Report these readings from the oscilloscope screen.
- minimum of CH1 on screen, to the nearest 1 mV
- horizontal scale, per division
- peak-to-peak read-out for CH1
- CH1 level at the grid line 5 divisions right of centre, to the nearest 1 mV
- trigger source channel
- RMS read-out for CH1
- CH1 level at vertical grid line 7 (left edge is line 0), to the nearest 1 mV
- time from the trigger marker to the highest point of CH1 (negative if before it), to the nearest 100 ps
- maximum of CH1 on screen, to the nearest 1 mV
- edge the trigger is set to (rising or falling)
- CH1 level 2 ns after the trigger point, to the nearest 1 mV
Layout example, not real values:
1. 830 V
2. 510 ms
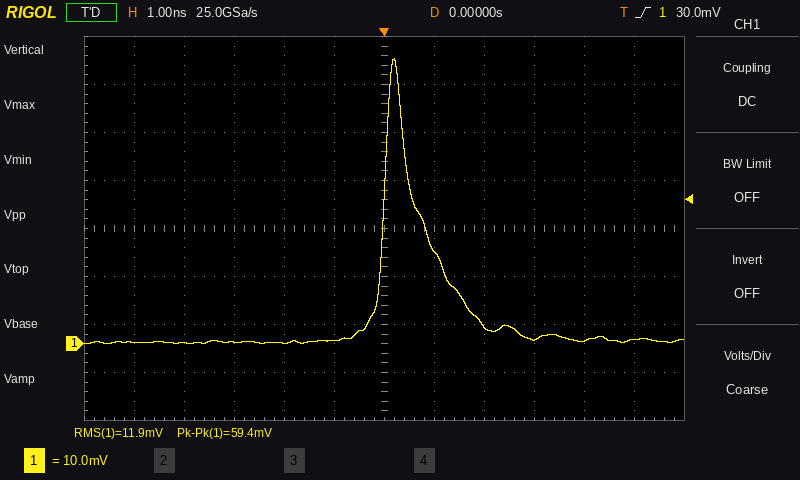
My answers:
1. 0 mV
2. 1 ns
3. 59.4 mV
4. 1 mV
5. CH1
6. 11.9 mV
7. 19 mV
8. +200 ps
9. 59 mV
10. rising
11. 4 mV
